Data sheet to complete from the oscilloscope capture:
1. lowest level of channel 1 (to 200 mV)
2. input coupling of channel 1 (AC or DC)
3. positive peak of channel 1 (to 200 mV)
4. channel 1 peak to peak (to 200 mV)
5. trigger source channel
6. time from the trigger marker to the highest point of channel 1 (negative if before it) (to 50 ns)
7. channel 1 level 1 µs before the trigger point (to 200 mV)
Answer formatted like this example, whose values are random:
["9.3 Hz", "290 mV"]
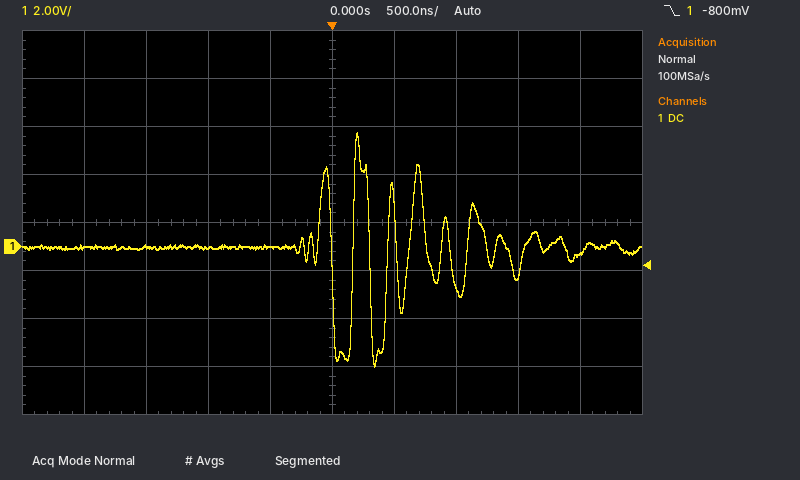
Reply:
["-5.0 V", "DC", "4.8 V", "9.8 V", "channel 1", "+200 ns", "0.0 V"]
